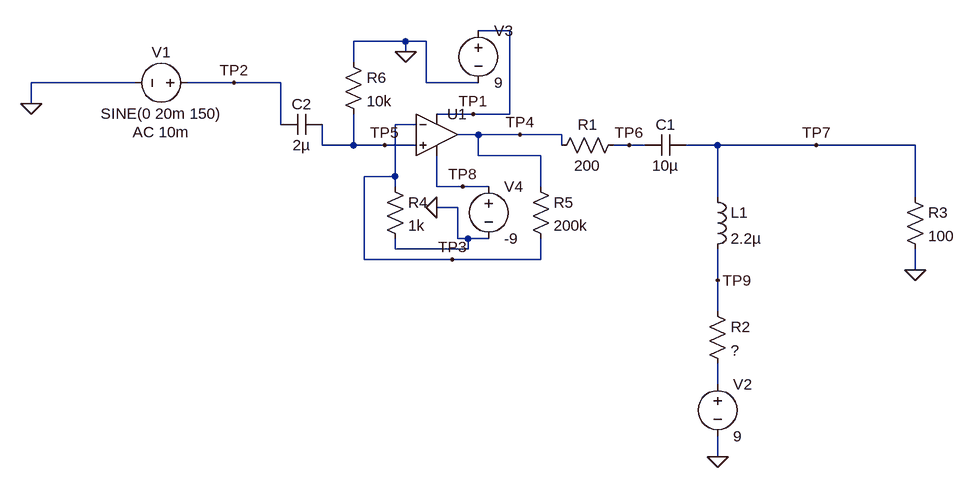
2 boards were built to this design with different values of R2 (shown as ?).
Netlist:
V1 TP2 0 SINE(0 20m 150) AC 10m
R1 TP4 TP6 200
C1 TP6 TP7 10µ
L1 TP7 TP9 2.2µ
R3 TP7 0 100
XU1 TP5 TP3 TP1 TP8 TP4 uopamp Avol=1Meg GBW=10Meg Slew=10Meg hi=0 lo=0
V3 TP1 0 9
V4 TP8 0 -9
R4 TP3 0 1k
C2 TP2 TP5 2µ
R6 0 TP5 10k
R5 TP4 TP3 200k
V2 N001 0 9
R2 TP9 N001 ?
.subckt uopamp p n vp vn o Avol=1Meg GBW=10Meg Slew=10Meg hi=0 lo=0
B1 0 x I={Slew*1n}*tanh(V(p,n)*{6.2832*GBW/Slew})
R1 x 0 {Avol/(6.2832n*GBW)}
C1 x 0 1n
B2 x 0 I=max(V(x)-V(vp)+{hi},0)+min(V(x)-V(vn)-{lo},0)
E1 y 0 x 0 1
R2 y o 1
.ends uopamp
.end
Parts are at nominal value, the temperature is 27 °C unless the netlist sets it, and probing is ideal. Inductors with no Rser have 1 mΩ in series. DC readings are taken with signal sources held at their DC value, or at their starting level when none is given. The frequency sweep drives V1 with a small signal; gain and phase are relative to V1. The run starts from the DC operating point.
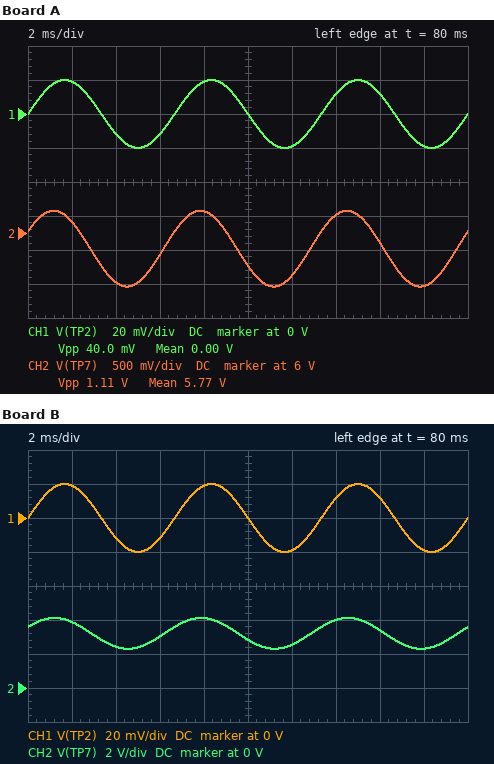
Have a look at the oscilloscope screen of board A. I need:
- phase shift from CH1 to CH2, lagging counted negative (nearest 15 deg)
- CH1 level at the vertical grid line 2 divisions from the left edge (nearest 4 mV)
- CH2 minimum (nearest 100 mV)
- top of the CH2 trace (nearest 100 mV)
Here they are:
30 deg
-12 mV
5.2 V
6.3 V
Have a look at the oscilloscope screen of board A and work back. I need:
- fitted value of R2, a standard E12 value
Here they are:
56 Ω
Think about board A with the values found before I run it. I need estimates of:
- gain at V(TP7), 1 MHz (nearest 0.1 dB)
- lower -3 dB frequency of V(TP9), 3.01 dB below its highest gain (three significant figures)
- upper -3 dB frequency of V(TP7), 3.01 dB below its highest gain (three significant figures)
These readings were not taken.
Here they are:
3.8 dB
68.2 Hz
49.7 kHz
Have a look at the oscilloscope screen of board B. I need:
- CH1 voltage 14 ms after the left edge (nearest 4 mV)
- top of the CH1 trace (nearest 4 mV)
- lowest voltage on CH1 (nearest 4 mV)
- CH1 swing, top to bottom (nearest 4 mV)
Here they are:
12 mV
20 mV
-20 mV
40 mV
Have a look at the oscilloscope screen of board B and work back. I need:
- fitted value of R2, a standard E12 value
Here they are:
180 Ω
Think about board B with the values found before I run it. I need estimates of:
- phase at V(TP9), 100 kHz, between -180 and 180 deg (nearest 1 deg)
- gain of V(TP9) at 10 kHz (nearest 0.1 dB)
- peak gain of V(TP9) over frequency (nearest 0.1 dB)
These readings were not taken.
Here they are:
-64 deg
33.6 dB
33.8 dB
